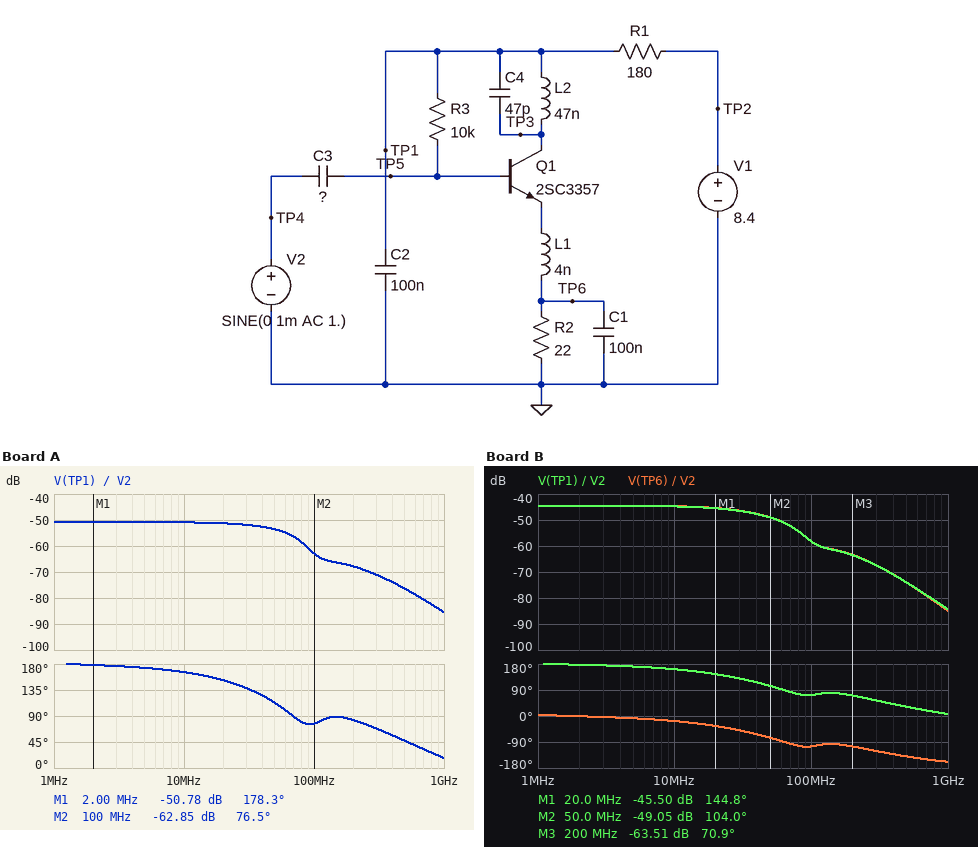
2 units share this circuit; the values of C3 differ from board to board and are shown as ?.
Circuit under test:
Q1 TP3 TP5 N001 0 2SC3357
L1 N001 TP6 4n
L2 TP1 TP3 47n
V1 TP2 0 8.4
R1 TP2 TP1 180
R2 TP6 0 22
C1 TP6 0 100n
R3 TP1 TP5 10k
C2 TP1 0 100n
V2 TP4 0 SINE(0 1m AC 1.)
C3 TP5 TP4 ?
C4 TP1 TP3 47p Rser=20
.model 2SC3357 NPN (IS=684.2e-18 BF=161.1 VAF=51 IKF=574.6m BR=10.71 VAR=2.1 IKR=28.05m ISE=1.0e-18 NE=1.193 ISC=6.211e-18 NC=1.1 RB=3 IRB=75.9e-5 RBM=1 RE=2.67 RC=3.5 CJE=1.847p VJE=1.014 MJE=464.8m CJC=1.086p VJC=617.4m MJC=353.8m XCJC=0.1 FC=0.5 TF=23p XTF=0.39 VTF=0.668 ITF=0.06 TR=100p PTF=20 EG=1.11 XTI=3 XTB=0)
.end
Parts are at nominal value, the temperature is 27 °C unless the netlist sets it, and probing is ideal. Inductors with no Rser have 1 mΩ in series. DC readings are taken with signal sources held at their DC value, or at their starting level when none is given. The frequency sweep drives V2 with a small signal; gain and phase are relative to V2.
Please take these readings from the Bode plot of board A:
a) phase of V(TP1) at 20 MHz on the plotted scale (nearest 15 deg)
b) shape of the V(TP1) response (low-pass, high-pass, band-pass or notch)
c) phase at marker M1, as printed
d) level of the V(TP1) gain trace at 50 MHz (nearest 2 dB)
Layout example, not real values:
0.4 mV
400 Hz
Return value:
150 deg
low-pass
178.3 deg
-54 dB
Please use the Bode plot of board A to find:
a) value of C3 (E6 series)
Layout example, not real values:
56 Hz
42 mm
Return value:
3.3 pF
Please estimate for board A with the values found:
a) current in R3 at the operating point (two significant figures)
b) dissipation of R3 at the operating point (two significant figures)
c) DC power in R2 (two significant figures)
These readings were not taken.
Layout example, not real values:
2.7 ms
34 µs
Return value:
250 µA
620 µW
14 mW
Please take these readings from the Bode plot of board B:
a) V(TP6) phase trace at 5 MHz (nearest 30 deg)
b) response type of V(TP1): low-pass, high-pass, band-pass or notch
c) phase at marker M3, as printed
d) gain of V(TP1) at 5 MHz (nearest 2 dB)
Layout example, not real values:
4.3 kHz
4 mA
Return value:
0 deg
low-pass
70.9 deg
-44 dB
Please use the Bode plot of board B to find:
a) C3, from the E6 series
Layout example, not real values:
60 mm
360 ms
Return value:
6.8 pF
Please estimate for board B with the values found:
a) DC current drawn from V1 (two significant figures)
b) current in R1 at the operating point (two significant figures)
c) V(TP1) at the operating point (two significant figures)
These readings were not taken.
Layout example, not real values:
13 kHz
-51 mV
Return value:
25 mA
25 mA
3.9 V
